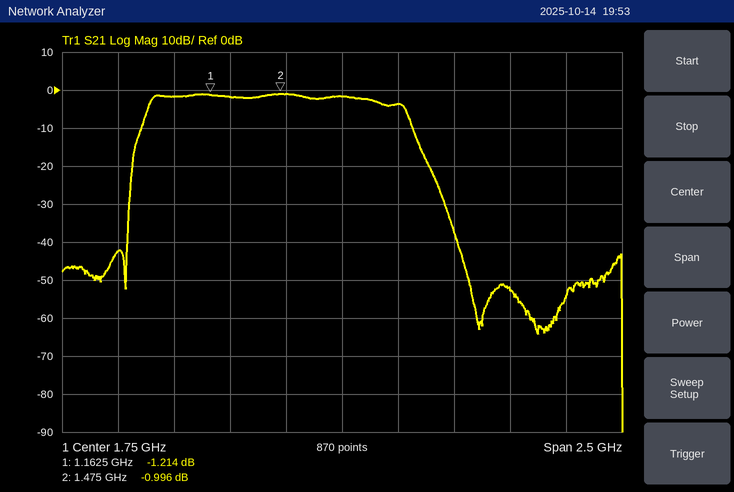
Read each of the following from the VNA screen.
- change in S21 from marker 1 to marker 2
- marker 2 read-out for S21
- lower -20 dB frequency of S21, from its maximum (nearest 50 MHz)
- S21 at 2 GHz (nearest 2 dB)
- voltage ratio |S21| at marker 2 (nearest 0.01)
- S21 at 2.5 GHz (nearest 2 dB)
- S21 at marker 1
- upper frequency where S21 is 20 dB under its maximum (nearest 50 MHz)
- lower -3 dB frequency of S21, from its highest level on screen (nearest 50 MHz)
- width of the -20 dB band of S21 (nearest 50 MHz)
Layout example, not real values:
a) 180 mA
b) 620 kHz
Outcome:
a) 0.218 dB
b) -0.996 dB
c) 800 MHz
d) -4 dB
e) 0.89
f) -52 dB
g) -1.214 dB
h) 2.15 GHz
i) 900 MHz
j) 1.35 GHz
